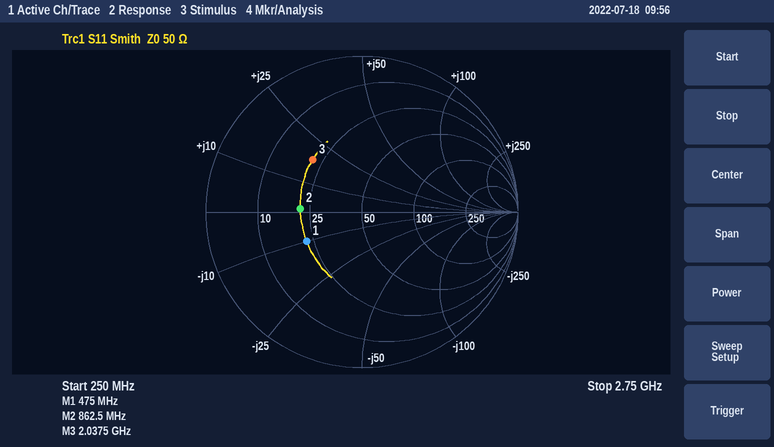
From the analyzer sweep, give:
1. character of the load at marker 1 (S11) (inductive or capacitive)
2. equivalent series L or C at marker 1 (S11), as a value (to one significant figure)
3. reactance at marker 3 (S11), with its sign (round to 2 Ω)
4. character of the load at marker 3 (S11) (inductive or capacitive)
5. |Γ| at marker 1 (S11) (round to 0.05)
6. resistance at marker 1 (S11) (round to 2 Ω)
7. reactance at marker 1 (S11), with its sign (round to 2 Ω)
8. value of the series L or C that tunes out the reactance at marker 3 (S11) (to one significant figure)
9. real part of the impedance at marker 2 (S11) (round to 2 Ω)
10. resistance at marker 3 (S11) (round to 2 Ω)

capacitive
30 pF
+18 Ω
inductive
0.40
22 Ω
-10 Ω
4 pF
22 Ω
22 Ω
